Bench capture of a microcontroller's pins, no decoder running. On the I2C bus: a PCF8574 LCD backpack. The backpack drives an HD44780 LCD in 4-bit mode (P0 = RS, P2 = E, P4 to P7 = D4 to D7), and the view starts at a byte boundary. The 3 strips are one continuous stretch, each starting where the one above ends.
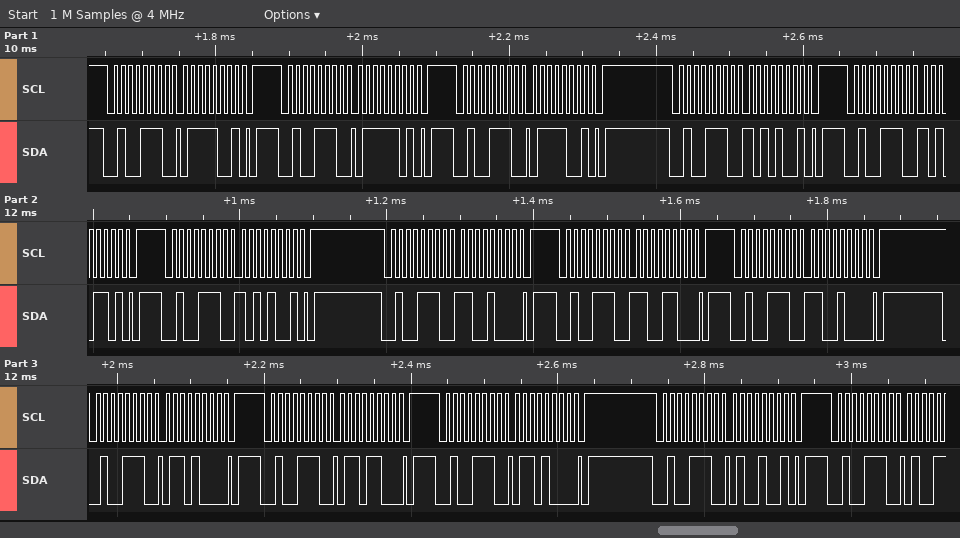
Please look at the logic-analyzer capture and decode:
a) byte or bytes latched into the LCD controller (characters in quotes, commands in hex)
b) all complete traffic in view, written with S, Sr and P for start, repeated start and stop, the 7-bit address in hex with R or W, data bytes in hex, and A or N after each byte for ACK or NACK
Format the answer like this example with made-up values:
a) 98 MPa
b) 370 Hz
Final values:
a) 'z' 0xC6
b) S 27W A 79 A P S 27W A 7D A P S 27W A 79 A P S 27W A A9 A P S 27W A AD A P S 27W A A9 A P S 27W A C8 A P S 27W A CC A P S 27W A C8 A P S 27W A 68 A P S 27W A 6C A P S 27W A 68 A P S 27W A 49 A P S 27W A
